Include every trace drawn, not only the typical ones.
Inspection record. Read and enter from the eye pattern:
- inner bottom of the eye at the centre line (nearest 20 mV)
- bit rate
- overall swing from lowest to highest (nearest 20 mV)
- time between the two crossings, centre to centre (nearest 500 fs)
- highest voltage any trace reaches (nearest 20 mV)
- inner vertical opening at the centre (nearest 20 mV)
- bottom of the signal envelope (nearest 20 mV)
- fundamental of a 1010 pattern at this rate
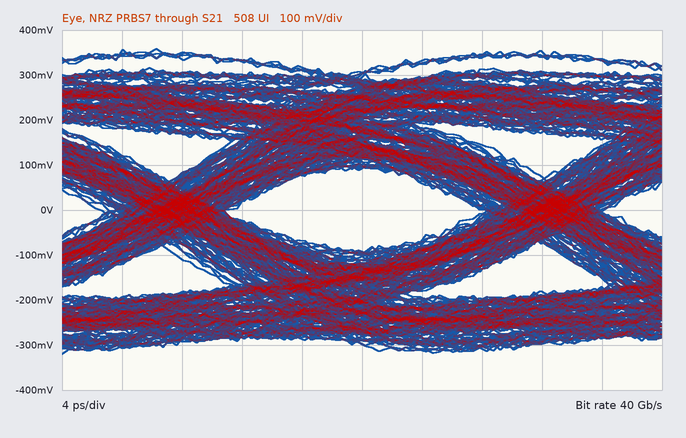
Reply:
-100 mV
40 Gb/s
680 mV
25.0 ps
360 mV
180 mV
-320 mV
20 GHz
